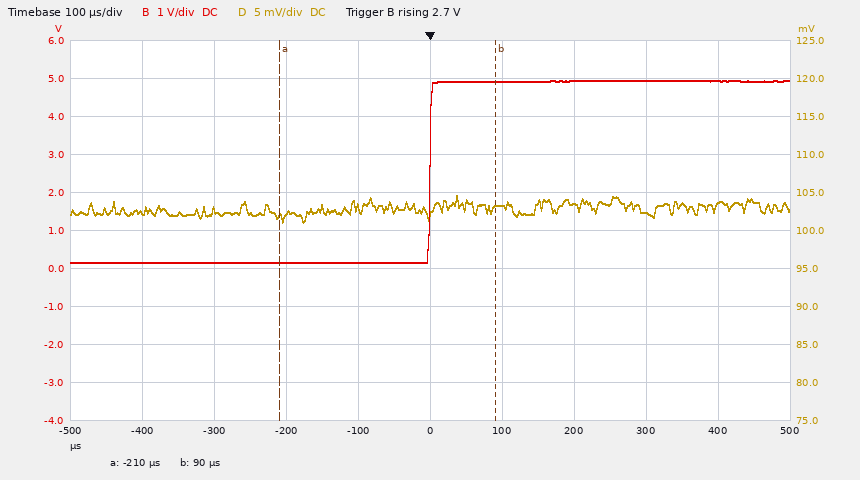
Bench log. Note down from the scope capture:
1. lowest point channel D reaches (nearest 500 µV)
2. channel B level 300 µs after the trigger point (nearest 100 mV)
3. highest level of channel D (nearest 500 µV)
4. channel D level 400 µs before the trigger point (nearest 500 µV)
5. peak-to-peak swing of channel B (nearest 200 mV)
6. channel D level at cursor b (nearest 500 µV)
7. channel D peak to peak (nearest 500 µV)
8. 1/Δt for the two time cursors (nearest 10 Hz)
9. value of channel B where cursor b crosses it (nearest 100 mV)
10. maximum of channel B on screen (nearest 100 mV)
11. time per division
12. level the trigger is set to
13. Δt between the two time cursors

101.0 mV
4.9 V
104.5 mV
102.5 mV
4.8 V
103.0 mV
3.5 mV
3.33 kHz
4.9 V
4.9 V
100 µs
2.7 V
300 µs
